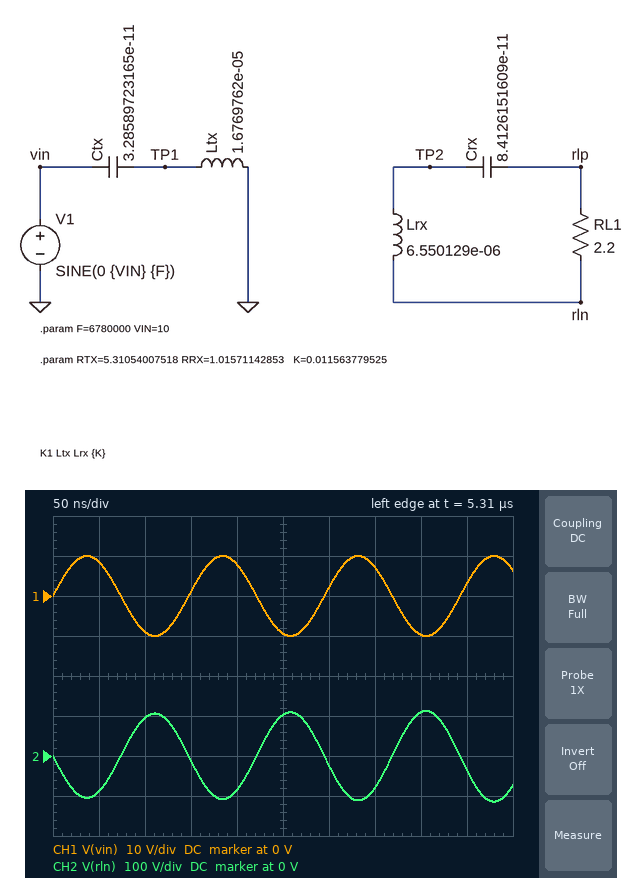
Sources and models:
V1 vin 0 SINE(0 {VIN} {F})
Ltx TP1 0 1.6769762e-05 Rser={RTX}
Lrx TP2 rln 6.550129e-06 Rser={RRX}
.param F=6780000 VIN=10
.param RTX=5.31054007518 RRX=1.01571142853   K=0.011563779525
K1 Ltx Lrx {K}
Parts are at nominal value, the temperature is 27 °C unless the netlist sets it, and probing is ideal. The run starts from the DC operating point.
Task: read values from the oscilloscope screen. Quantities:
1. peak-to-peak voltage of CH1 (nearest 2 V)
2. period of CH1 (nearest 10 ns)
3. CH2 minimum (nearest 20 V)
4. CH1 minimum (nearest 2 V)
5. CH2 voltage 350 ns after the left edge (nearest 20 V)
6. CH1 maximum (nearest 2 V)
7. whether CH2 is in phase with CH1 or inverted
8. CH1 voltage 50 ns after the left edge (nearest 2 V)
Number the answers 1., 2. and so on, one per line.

1. 20 V
2. 150 ns
3. -120 V
4. -10 V
5. -80 V
6. 10 V
7. inverted
8. 8 V
